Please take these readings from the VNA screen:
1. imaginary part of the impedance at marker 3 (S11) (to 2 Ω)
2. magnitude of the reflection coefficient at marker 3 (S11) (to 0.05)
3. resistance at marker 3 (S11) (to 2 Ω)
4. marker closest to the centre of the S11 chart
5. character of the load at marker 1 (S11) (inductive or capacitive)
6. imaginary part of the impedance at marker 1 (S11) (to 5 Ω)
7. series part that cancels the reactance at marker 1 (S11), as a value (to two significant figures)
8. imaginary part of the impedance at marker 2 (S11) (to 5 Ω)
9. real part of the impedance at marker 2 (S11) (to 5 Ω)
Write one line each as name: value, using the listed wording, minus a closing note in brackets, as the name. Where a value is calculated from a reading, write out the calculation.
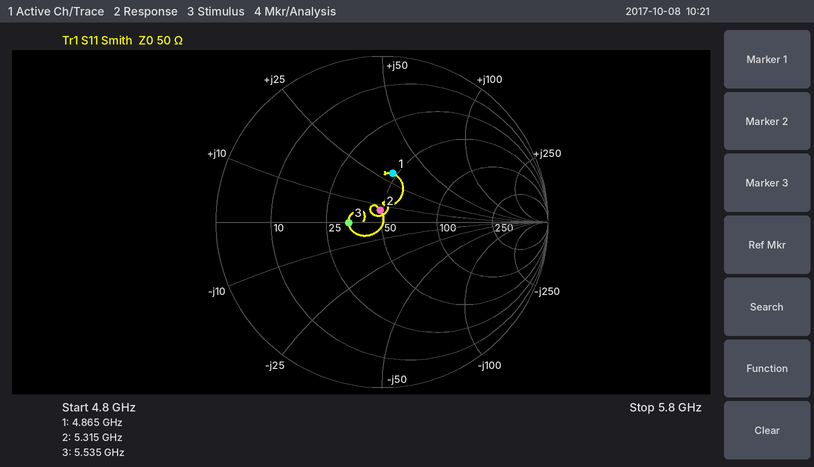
imaginary part of the impedance at marker 3 (S11): 0 Ω
magnitude of the reflection coefficient at marker 3 (S11): 0.20
resistance at marker 3 (S11): 34 Ω
marker closest to the centre of the S11 chart: marker 2
character of the load at marker 1 (S11): inductive
imaginary part of the impedance at marker 1 (S11): +30 Ω
series part that cancels the reactance at marker 1 (S11), as a value: C = 1/(2π × 4.865 GHz × 30 Ω) ≈ 1.1 pF
imaginary part of the impedance at marker 2 (S11): +5 Ω
real part of the impedance at marker 2 (S11): 50 Ω
